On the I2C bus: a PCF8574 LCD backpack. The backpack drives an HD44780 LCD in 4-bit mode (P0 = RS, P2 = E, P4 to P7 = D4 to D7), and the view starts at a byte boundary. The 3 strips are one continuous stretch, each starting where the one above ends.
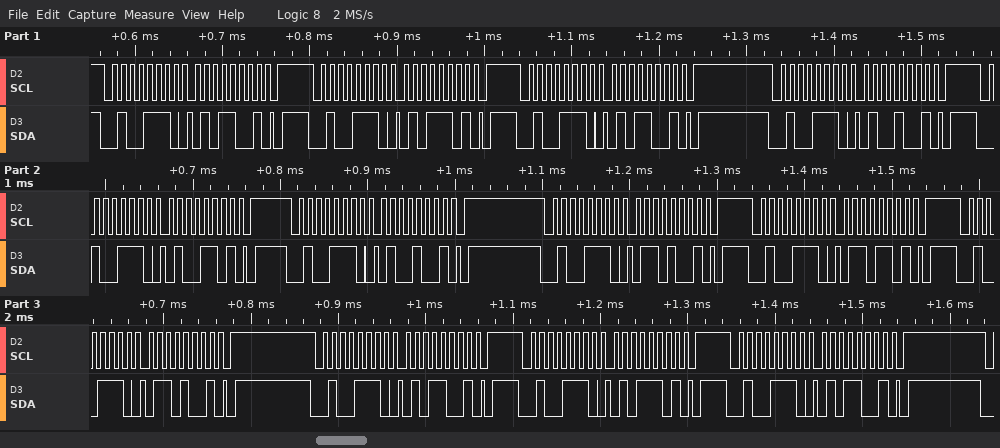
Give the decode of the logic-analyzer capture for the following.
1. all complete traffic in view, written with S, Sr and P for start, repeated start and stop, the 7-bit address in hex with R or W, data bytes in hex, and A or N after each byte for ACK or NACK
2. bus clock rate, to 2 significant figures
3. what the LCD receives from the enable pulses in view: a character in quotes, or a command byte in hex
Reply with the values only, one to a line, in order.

S 27W A 59 A P S 27W A 5D A P S 27W A 59 A P S 27W A 49 A P S 27W A 4D A P S 27W A 49 A P S 27W A 69 A P S 27W A 6D A P S 27W A 69 A P S 27W A 59 A P S 27W A 5D A P S 27W A 59 A P
100 kHz
'T' 'e'
